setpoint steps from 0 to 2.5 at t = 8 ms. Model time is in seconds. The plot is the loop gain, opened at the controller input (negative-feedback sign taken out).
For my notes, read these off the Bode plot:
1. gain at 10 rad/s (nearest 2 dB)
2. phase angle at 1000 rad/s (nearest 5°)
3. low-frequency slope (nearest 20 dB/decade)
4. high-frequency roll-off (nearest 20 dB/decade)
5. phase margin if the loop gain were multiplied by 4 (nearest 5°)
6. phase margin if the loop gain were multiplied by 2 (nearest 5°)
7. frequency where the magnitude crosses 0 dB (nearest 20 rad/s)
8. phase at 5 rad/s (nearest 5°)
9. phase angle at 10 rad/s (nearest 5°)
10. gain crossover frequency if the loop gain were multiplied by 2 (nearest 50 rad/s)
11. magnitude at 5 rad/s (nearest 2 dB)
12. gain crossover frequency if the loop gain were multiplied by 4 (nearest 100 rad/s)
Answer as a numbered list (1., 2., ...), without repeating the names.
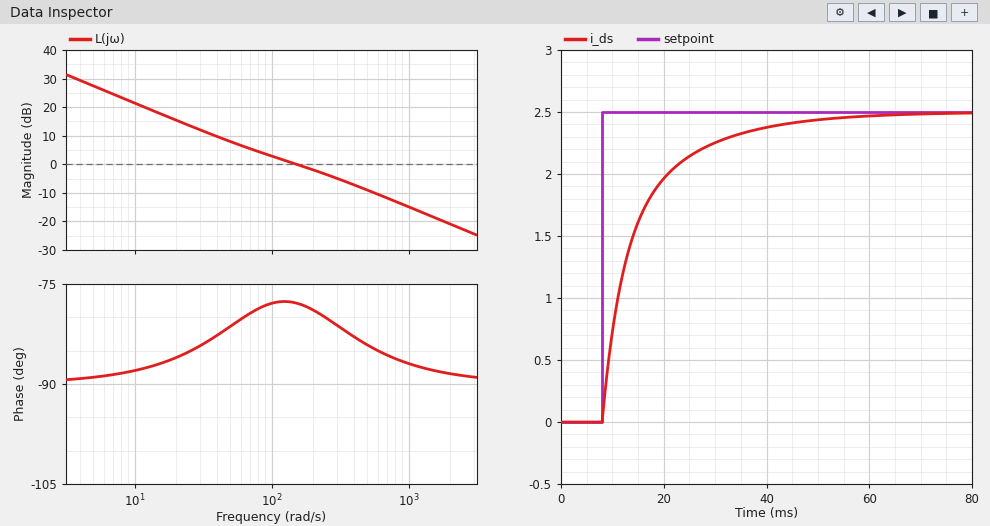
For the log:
1. 22 dB
2. -85°
3. -20 dB/decade
4. -20 dB/decade
5. 95°
6. 100°
7. 160 rad/s
8. -90°
9. -90°
10. 350 rad/s
11. 28 dB
12. 700 rad/s
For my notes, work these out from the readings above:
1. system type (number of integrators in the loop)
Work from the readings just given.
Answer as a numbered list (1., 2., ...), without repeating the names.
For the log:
1. 1
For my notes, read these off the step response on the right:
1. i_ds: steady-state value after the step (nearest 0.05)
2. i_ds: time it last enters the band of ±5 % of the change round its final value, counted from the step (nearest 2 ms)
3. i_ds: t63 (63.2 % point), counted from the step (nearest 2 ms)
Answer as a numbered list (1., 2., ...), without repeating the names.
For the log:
1. 2.50
2. 32 ms
3. 6 ms
